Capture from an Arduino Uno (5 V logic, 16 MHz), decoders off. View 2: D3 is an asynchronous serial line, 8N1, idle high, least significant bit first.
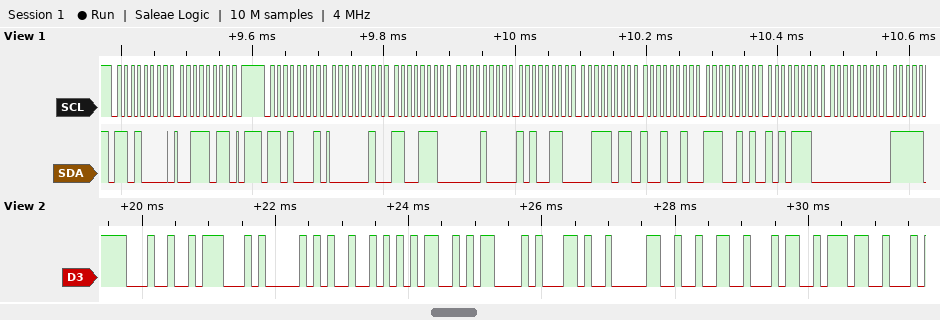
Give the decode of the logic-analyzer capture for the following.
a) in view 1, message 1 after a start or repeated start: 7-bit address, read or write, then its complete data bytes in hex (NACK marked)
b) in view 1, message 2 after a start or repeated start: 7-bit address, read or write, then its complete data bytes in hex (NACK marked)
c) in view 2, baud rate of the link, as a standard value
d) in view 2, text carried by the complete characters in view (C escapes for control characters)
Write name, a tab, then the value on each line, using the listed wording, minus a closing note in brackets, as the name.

in view 1, message 1 after a start or repeated start: 7-bit address, read or write, then its complete data bytes in hex	0x68 write: 3B
in view 1, message 2 after a start or repeated start: 7-bit address, read or write, then its complete data bytes in hex	0x68 read: 02 CE 08 A6 3B 92 E5 AE 00
in view 2, baud rate of the link, as a standard value	9600 baud
in view 2, text carried by the complete characters in view	"$GPRMC,0247"
